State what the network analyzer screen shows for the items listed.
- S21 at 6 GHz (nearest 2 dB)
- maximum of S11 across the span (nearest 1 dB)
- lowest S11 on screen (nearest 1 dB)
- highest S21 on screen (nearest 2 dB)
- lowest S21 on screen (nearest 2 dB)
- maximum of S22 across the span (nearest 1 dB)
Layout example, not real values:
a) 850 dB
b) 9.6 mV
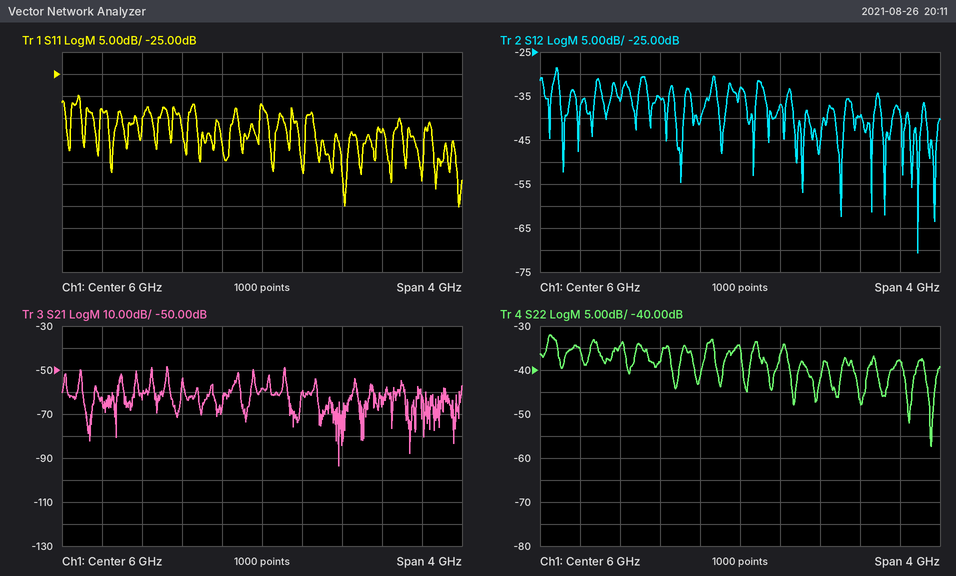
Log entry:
a) -58 dB
b) -30 dB
c) -55 dB
d) -48 dB
e) -94 dB
f) -32 dB
